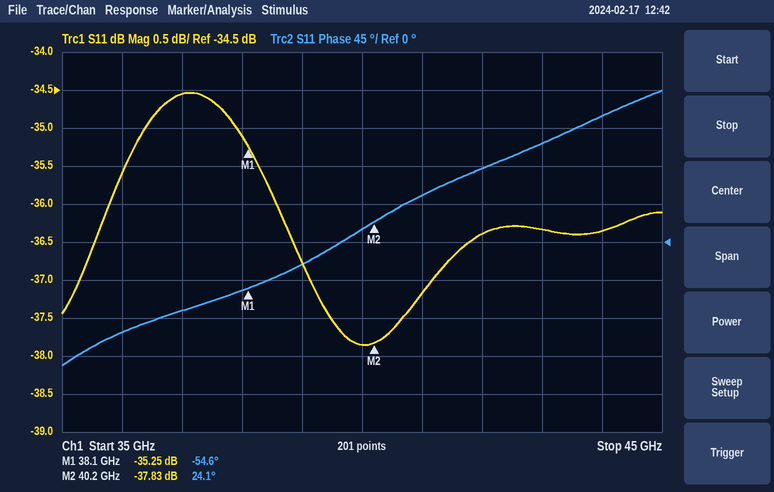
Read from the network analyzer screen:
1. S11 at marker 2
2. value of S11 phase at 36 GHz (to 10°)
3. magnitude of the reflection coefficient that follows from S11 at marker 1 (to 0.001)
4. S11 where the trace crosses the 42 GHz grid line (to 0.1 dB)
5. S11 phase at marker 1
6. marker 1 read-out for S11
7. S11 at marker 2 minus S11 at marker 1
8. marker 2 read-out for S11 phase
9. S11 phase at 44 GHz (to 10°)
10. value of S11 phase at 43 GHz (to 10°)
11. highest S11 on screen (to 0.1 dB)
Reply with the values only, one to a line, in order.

-37.83 dB
-110°
0.017
-36.4 dB
-54.6°
-35.25 dB
-2.58 dB
24.1°
150°
120°
-34.5 dB
